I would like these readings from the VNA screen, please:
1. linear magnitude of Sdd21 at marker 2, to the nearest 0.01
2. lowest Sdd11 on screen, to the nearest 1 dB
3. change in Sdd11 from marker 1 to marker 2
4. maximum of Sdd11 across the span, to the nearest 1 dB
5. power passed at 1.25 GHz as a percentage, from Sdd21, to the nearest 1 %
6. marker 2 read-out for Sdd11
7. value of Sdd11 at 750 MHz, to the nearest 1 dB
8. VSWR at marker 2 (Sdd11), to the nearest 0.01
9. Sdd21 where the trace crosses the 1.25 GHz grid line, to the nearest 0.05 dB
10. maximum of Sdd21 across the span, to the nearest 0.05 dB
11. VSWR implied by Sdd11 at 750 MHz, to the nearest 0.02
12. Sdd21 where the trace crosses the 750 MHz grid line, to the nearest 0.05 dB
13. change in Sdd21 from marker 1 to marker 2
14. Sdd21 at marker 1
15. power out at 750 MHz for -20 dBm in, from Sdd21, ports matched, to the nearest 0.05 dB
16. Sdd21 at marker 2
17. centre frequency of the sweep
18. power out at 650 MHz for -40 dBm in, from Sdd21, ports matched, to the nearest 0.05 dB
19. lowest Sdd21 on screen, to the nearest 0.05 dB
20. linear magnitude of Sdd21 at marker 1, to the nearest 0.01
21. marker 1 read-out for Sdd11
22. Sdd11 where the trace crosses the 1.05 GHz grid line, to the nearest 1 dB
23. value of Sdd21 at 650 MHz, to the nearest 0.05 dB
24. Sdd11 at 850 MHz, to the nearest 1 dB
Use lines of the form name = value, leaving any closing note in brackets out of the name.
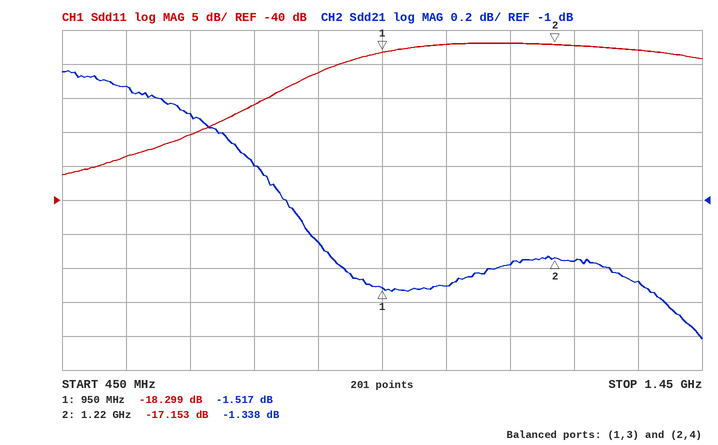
linear magnitude of Sdd21 at marker 2, to the nearest 0.01 = 0.86
lowest Sdd11 on screen, to the nearest 1 dB = -36 dB
change in Sdd11 from marker 1 to marker 2 = 1.146 dB
maximum of Sdd11 across the span, to the nearest 1 dB = -17 dB
power passed at 1.25 GHz as a percentage, from Sdd21, to the nearest 1 % = 73 %
marker 2 read-out for Sdd11 = -17.153 dB
value of Sdd11 at 750 MHz, to the nearest 1 dB = -26 dB
VSWR at marker 2 (Sdd11), to the nearest 0.01 = 1.32
Sdd21 where the trace crosses the 1.25 GHz grid line, to the nearest 0.05 dB = -1.35 dB
maximum of Sdd21 across the span, to the nearest 0.05 dB = -0.25 dB
VSWR implied by Sdd11 at 750 MHz, to the nearest 0.02 = 1.10
Sdd21 where the trace crosses the 750 MHz grid line, to the nearest 0.05 dB = -0.80 dB
change in Sdd21 from marker 1 to marker 2 = 0.179 dB
Sdd21 at marker 1 = -1.517 dB
power out at 750 MHz for -20 dBm in, from Sdd21, ports matched, to the nearest 0.05 dB = -20.80 dBm
Sdd21 at marker 2 = -1.338 dB
centre frequency of the sweep = 950 MHz
power out at 650 MHz for -40 dBm in, from Sdd21, ports matched, to the nearest 0.05 dB = -40.50 dBm
lowest Sdd21 on screen, to the nearest 0.05 dB = -1.80 dB
linear magnitude of Sdd21 at marker 1, to the nearest 0.01 = 0.84
marker 1 read-out for Sdd11 = -18.299 dB
Sdd11 where the trace crosses the 1.05 GHz grid line, to the nearest 1 dB = -17 dB
value of Sdd21 at 650 MHz, to the nearest 0.05 dB = -0.50 dB
Sdd11 at 850 MHz, to the nearest 1 dB = -21 dB
